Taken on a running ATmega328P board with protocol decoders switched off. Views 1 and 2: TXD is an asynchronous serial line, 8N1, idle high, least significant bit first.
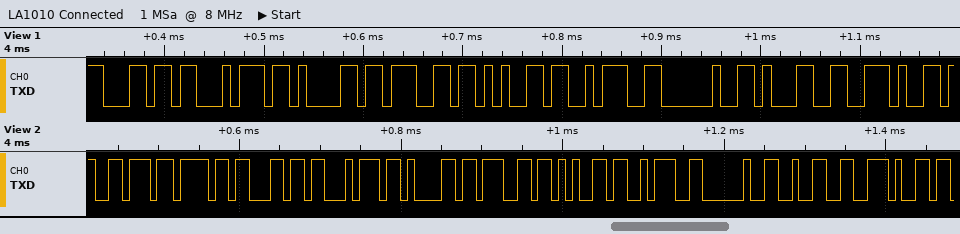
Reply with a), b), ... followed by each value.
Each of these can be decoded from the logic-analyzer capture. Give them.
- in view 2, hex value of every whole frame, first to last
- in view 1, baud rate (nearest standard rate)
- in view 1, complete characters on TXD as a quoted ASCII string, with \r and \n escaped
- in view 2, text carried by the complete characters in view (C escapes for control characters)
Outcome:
a) 0x76 0x6F 0x6C 0x74 0x61 0x67 0x65 0x3A 0x20 0x32 0x2E
b) 115200 baud
c) "ltage: 1."
d) "voltage: 2."
